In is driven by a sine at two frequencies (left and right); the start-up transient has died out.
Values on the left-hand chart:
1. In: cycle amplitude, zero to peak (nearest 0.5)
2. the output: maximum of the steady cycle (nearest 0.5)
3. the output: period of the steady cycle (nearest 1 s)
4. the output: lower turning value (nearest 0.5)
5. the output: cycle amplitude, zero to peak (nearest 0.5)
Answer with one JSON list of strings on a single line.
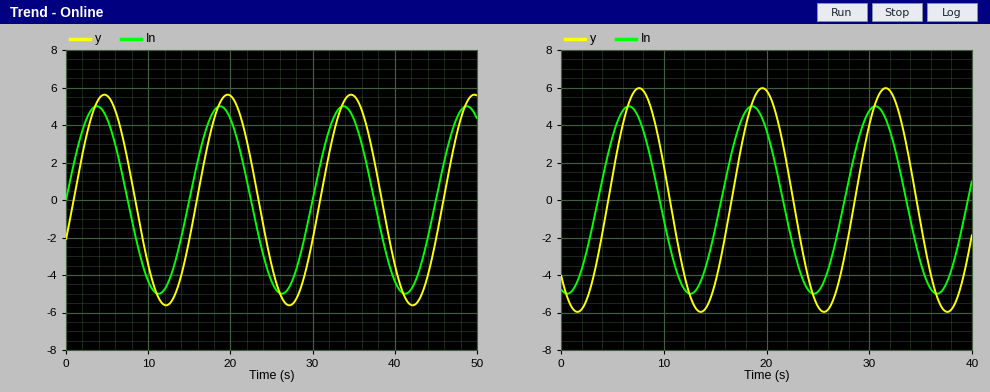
["5.0", "5.5", "15 s", "-5.5", "5.5"]
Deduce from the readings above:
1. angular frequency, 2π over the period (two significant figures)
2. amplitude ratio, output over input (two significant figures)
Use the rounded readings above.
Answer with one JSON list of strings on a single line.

["0.42 rad/s", "1.1"]
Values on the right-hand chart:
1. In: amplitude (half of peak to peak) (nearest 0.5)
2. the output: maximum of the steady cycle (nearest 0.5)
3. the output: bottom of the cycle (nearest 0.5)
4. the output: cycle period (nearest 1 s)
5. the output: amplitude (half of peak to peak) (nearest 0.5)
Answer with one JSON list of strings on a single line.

["5.0", "6.0", "-6.0", "12 s", "6.0"]
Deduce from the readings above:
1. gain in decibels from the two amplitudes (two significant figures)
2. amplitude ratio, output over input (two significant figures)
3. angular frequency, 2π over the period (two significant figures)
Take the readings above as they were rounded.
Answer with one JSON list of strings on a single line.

["1.6 dB", "1.2", "0.52 rad/s"]
